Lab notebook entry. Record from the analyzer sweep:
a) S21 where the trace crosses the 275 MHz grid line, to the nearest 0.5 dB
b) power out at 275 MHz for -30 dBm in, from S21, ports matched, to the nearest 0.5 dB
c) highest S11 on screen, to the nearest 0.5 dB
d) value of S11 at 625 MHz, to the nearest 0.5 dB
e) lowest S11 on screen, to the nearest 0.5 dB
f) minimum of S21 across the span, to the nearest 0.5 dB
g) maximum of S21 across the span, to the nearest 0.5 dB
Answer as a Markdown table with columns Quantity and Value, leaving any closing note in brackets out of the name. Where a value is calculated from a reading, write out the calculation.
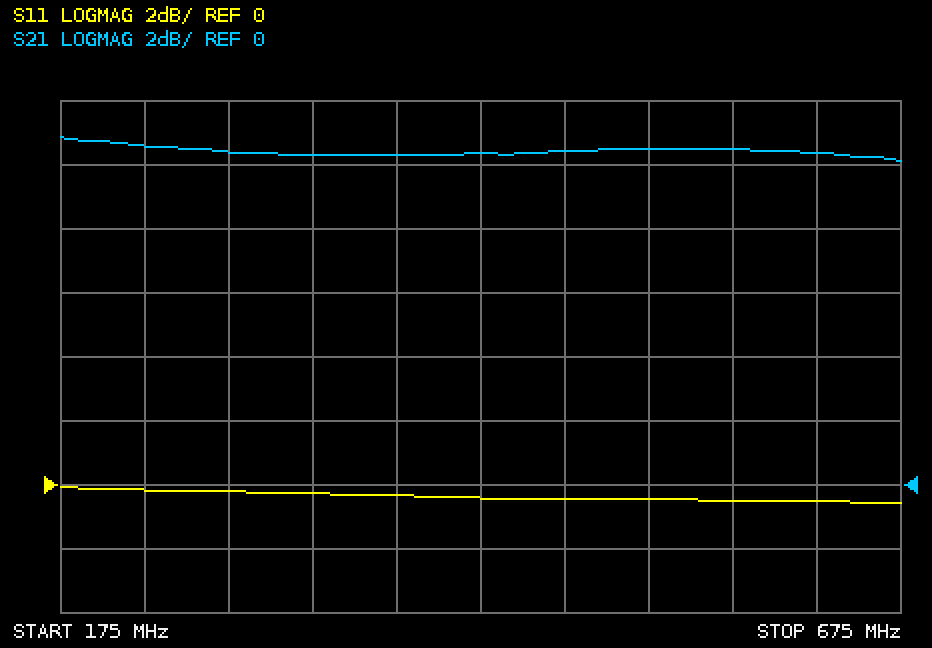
| Quantity | Value |
|---|---|
| S21 where the trace crosses the 275 MHz grid line, to the nearest 0.5 dB | 10.5 dB |
| power out at 275 MHz for -30 dBm in, from S21, ports matched, to the nearest 0.5 dB | -30 dBm + (10.5 dB) = -19.5 dBm |
| highest S11 on screen, to the nearest 0.5 dB | 0.0 dB |
| value of S11 at 625 MHz, to the nearest 0.5 dB | -0.5 dB |
| lowest S11 on screen, to the nearest 0.5 dB | -0.5 dB |
| minimum of S21 across the span, to the nearest 0.5 dB | 10.0 dB |
| maximum of S21 across the span, to the nearest 0.5 dB | 11.0 dB |
